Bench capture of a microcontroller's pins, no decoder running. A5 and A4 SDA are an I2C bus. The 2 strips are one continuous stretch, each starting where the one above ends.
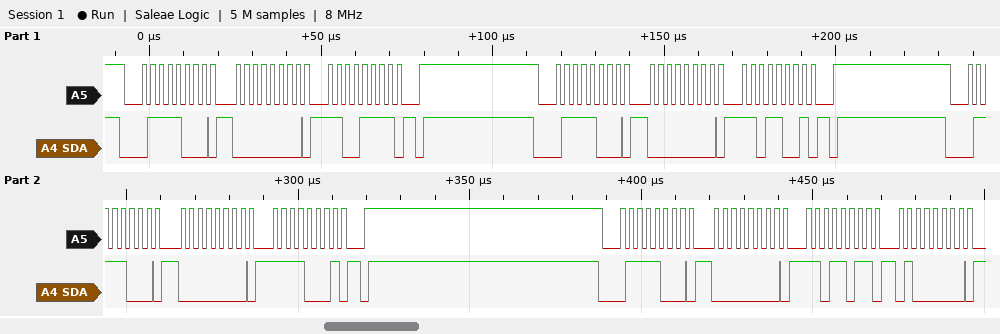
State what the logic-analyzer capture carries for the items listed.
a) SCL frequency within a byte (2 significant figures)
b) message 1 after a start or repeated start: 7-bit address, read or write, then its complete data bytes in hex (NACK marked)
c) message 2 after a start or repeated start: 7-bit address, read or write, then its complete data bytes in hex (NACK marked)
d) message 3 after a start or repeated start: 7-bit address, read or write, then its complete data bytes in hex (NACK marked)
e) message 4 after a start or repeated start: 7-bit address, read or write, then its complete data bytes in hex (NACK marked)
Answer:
400 kHz
0x3C write: 00 CF
0x3C write: 00 D9
0x3C write: 00 F1
0x3C write: 00 DB 40
